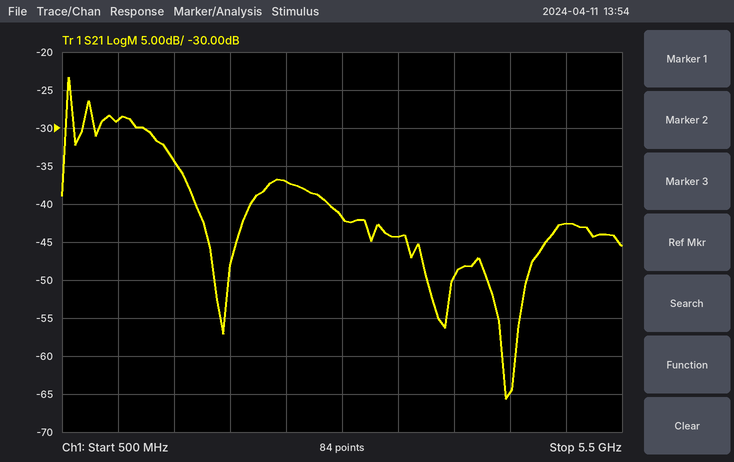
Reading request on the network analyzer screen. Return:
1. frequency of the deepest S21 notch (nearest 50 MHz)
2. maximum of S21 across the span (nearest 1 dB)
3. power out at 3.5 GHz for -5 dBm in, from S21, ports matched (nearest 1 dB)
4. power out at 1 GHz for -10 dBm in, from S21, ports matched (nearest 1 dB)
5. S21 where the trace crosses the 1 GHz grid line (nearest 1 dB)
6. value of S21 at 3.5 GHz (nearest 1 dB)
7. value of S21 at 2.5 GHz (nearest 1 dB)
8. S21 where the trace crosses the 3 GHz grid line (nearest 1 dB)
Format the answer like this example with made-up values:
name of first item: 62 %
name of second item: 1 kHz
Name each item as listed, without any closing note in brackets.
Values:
frequency of the deepest S21 notch: 4.45 GHz
maximum of S21 across the span: -23 dB
power out at 3.5 GHz for -5 dBm in, from S21, ports matched: -49 dBm
power out at 1 GHz for -10 dBm in, from S21, ports matched: -39 dBm
S21 where the trace crosses the 1 GHz grid line: -29 dB
value of S21 at 3.5 GHz: -44 dB
value of S21 at 2.5 GHz: -37 dB
S21 where the trace crosses the 3 GHz grid line: -42 dB
